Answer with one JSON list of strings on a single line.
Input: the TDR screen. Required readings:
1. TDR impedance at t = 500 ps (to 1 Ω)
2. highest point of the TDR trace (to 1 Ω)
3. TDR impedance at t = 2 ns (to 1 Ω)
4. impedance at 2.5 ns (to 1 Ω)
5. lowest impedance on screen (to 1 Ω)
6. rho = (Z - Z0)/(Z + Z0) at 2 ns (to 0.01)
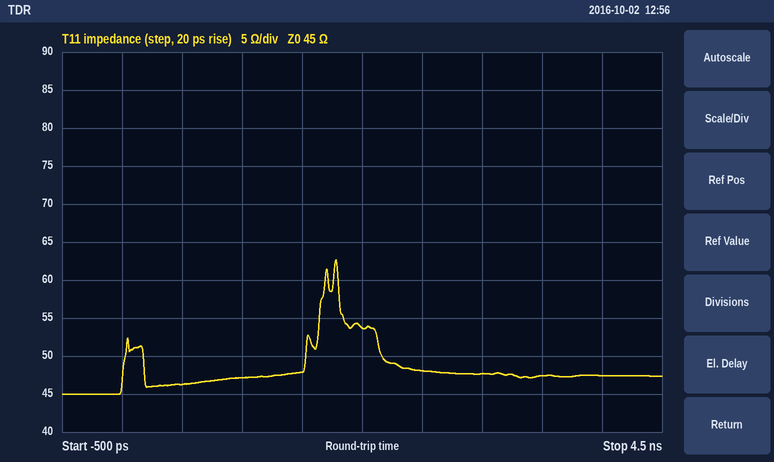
["46 Ω", "63 Ω", "54 Ω", "48 Ω", "45 Ω", "+0.09"]
